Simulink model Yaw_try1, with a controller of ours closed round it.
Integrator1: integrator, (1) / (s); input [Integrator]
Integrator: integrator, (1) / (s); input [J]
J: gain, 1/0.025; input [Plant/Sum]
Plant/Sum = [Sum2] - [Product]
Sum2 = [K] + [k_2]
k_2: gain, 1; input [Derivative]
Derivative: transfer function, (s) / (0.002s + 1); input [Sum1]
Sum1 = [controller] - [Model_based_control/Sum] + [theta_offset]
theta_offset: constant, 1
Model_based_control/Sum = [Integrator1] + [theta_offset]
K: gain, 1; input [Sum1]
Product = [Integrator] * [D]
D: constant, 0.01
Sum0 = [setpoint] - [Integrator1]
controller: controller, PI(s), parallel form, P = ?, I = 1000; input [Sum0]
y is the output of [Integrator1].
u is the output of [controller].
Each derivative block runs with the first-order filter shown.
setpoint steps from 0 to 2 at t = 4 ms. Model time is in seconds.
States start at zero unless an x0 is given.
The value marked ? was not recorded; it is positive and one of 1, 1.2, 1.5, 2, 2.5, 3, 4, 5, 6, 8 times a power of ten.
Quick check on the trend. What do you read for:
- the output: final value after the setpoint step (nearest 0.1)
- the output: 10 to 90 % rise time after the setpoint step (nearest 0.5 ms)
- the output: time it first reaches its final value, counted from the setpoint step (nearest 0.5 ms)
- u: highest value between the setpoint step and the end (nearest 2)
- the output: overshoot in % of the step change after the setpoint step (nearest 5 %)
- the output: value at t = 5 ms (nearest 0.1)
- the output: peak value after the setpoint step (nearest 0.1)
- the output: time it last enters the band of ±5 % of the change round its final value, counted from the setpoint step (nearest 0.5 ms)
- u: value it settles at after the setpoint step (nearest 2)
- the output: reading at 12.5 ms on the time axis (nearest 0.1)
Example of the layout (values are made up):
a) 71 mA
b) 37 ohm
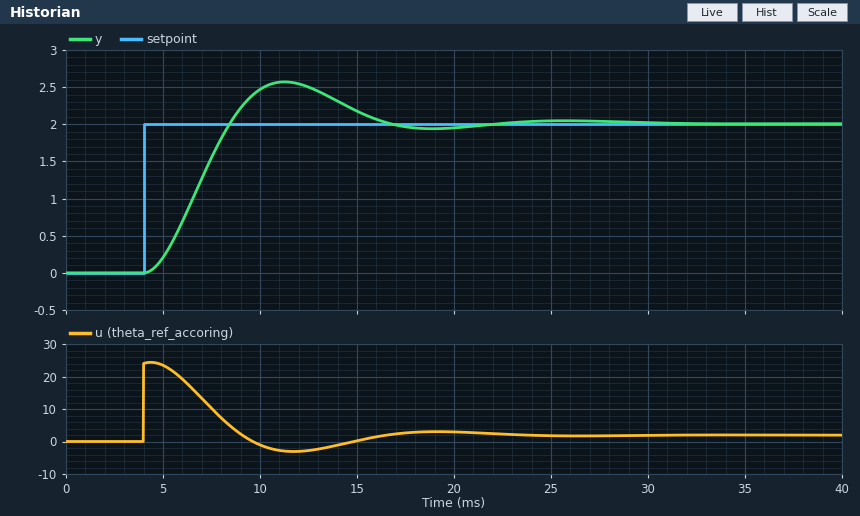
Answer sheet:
a) 2.0
b) 3.0 ms
c) 4.5 ms
d) 24
e) 30 %
f) 0.2
g) 2.6
h) 11.5 ms
i) 2
j) 2.5
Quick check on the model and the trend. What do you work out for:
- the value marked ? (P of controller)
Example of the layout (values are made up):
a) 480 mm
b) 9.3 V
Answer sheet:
a) 12
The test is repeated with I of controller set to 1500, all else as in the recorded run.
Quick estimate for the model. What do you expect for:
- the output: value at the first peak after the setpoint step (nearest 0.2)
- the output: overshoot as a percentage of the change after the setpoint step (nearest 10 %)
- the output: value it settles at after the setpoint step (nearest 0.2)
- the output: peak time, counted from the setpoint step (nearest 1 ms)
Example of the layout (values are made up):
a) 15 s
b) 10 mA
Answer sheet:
a) 2.8
b) 40 %
c) 2.0
d) 7 ms
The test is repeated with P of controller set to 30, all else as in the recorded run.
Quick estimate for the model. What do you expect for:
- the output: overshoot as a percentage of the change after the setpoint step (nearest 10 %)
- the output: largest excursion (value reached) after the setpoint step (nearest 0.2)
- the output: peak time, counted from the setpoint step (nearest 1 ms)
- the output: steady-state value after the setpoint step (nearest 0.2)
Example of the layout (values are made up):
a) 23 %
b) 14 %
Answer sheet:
a) 40 %
b) 2.8
c) 4 ms
d) 2.0
